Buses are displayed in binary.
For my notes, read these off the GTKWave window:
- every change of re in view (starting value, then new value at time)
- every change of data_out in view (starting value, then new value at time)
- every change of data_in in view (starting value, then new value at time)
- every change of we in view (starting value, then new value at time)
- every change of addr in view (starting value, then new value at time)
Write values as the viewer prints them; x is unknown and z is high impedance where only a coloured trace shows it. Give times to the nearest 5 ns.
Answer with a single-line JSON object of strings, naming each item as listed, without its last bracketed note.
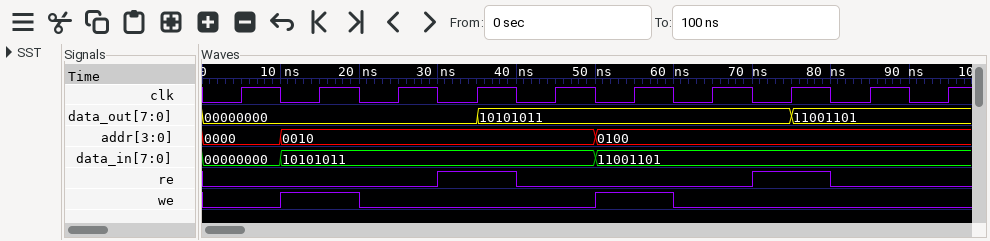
{"every change of re in view": "0, 1 at 30 ns, 0 at 40 ns, 1 at 70 ns, 0 at 80 ns", "every change of data_out in view": "00000000, 10101011 at 35 ns, 11001101 at 75 ns", "every change of data_in in view": "00000000, 10101011 at 10 ns, 11001101 at 50 ns", "every change of we in view": "0, 1 at 10 ns, 0 at 20 ns, 1 at 50 ns, 0 at 60 ns", "every change of addr in view": "0000, 0010 at 10 ns, 0100 at 50 ns"}
